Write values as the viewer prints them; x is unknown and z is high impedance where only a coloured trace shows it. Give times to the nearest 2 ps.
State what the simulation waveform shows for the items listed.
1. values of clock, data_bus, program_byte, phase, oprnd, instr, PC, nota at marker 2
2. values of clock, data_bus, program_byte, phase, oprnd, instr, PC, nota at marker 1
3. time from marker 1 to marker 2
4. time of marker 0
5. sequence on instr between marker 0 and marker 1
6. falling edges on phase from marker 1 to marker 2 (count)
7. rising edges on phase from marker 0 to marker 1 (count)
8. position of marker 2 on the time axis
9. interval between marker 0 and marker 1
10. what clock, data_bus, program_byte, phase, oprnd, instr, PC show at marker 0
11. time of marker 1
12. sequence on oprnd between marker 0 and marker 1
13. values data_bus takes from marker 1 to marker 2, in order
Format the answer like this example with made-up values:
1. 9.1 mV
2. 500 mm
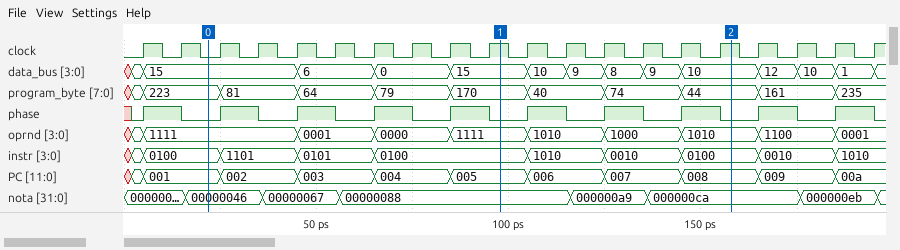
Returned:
1. clock=1, data_bus=10, program_byte=44, phase=0, oprnd=1010, instr=0100, PC=008, nota=000000ca
2. clock=1, data_bus=15, program_byte=170, phase=0, oprnd=1111, instr=0100, PC=005, nota=00000088
3. 60 ps
4. 22 ps
5. 0100, 1101, 0101, 0100
6. 3
7. 4
8. 158 ps
9. 76 ps
10. clock=0, data_bus=15, program_byte=223, phase=0, oprnd=1111, instr=0100, PC=001
11. 98 ps
12. 1111, 0001, 0000, 1111
13. 15, 10, 9, 8, 9, 10
